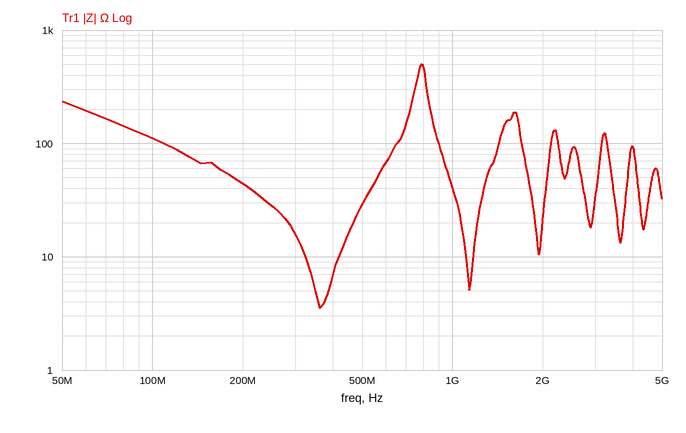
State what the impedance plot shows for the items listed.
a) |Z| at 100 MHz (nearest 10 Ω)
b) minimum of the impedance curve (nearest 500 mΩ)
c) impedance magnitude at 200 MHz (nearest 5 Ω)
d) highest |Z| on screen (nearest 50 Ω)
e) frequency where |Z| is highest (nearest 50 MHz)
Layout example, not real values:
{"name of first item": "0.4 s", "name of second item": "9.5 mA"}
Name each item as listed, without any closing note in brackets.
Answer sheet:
{"|Z| at 100 MHz": "110 Ω", "minimum of the impedance curve": "3.5 Ω", "impedance magnitude at 200 MHz": "45 Ω", "highest |Z| on screen": "500 Ω", "frequency where |Z| is highest": "800 MHz"}
